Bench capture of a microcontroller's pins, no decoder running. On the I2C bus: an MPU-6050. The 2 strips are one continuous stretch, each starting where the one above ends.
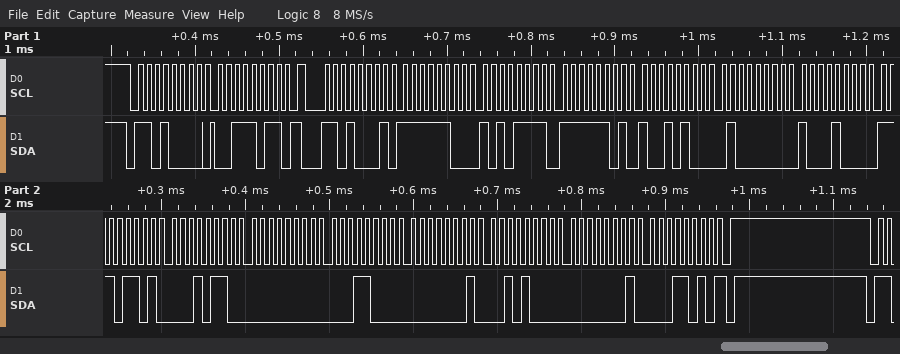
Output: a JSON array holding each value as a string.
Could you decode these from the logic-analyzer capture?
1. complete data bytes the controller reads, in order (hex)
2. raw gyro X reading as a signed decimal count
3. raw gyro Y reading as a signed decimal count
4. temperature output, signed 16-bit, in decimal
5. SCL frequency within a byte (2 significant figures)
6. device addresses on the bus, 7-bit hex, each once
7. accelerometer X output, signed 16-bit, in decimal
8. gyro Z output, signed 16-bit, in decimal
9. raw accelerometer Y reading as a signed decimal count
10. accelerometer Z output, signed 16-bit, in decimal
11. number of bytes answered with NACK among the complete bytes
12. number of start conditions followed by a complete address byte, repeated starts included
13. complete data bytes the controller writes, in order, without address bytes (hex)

["FC AF FD 94 40 88 ED 16 00 18 01 28 01 1A", "24", "296", "-4842", "100 kHz", "0x68", "-849", "282", "-620", "16520", "1", "2", "3B"]
